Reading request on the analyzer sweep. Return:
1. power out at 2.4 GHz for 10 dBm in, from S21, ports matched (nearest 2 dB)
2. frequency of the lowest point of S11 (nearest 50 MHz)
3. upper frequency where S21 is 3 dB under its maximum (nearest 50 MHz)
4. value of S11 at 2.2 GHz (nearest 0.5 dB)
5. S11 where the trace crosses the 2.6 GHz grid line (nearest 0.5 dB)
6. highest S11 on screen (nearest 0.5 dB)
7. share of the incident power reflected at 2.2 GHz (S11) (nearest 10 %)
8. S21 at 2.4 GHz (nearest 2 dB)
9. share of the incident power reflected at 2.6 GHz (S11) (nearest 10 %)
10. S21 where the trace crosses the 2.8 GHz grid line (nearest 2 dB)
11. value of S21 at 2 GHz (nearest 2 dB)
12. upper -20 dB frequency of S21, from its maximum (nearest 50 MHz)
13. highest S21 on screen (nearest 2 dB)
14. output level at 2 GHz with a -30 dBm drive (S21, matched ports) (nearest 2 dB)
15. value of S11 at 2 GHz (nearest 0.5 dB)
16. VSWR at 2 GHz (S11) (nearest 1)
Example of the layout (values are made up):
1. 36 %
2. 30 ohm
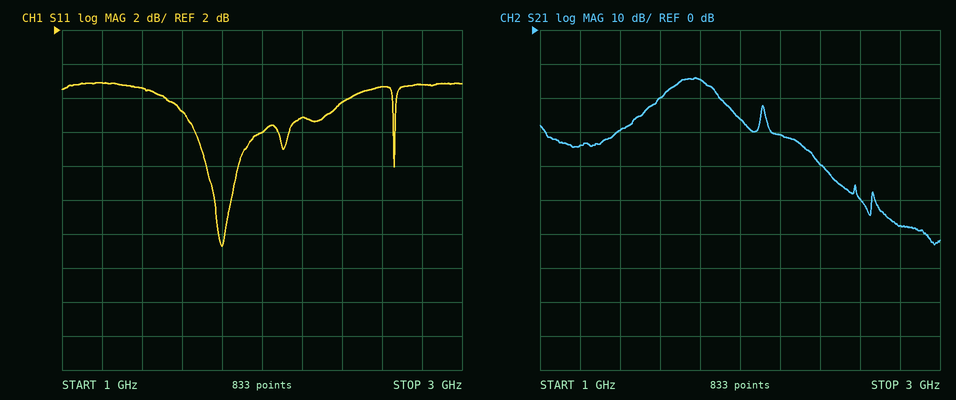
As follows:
1. -30 dBm
2. 1.80 GHz
3. 1.85 GHz
4. -3.0 dB
5. -1.5 dB
6. -1.0 dB
7. 50 %
8. -40 dB
9. 70 %
10. -58 dB
11. -26 dB
12. 2.30 GHz
13. -14 dB
14. -56 dBm
15. -4.0 dB
16. 4
